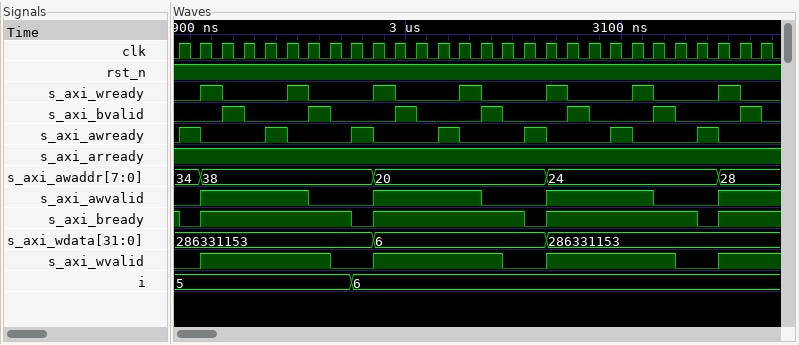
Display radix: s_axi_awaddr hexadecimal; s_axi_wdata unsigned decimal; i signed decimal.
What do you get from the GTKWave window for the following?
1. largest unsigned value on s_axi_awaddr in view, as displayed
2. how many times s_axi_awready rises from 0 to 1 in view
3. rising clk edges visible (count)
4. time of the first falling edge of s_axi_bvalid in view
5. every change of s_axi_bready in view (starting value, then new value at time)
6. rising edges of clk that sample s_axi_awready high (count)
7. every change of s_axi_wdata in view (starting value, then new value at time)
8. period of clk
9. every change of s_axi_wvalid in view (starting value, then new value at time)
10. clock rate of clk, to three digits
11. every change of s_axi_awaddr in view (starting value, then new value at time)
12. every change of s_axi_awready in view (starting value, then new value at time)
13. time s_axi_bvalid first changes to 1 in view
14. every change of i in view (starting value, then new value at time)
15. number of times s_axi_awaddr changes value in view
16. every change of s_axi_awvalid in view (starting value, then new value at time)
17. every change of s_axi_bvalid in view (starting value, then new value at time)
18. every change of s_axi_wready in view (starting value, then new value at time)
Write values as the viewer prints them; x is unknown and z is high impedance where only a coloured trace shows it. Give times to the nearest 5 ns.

38
7
28
2925 ns
1, 0 at 2895 ns, 1 at 2905 ns, 0 at 2975 ns, 1 at 2985 ns, 0 at 3055 ns, 1 at 3065 ns, 0 at 3135 ns, 1 at 3145 ns
7
286331153, 6 at 2985 ns, 286331153 at 3065 ns
10 ns
0, 1 at 2905 ns, 0 at 2965 ns, 1 at 2985 ns, 0 at 3045 ns, 1 at 3065 ns, 0 at 3125 ns, 1 at 3145 ns
100 MHz
34, 38 at 2905 ns, 20 at 2985 ns, 24 at 3065 ns, 28 at 3145 ns
0, 1 at 2895 ns, 0 at 2905 ns, 1 at 2935 ns, 0 at 2945 ns, 1 at 2975 ns, 0 at 2985 ns, 1 at 3015 ns, 0 at 3025 ns, 1 at 3055 ns, 0 at 3065 ns, 1 at 3095 ns, 0 at 3105 ns, 1 at 3135 ns, 0 at 3145 ns
2915 ns
5, 6 at 2975 ns
4
0, 1 at 2905 ns, 0 at 2955 ns, 1 at 2985 ns, 0 at 3035 ns, 1 at 3065 ns, 0 at 3115 ns, 1 at 3145 ns
0, 1 at 2915 ns, 0 at 2925 ns, 1 at 2955 ns, 0 at 2965 ns, 1 at 2995 ns, 0 at 3005 ns, 1 at 3035 ns, 0 at 3045 ns, 1 at 3075 ns, 0 at 3085 ns, 1 at 3115 ns, 0 at 3125 ns, 1 at 3155 ns, 0 at 3165 ns
0, 1 at 2905 ns, 0 at 2915 ns, 1 at 2945 ns, 0 at 2955 ns, 1 at 2985 ns, 0 at 2995 ns, 1 at 3025 ns, 0 at 3035 ns, 1 at 3065 ns, 0 at 3075 ns, 1 at 3105 ns, 0 at 3115 ns, 1 at 3145 ns, 0 at 3155 ns
